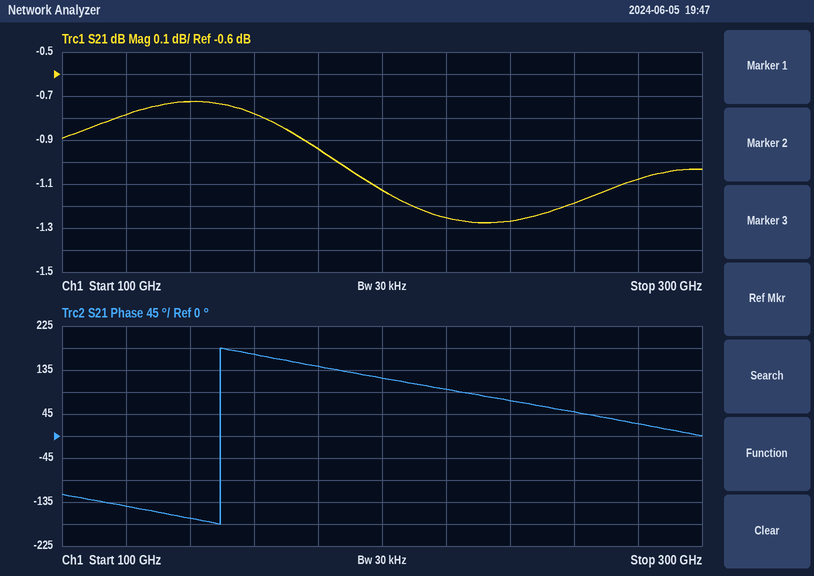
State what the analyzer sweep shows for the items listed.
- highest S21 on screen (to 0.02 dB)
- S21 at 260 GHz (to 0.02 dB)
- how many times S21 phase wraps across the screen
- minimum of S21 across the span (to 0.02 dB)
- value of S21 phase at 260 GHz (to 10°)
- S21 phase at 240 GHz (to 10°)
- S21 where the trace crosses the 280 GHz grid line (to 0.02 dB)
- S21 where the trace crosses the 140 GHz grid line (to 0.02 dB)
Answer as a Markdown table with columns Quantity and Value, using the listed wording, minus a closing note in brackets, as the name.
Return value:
| Quantity | Value |
|---|---|
| highest S21 on screen | -0.72 dB |
| S21 at 260 GHz | -1.18 dB |
| how many times S21 phase wraps across the screen | 1 |
| minimum of S21 across the span | -1.28 dB |
| value of S21 phase at 260 GHz | 50° |
| S21 phase at 240 GHz | 70° |
| S21 where the trace crosses the 280 GHz grid line | -1.08 dB |
| S21 where the trace crosses the 140 GHz grid line | -0.72 dB |
